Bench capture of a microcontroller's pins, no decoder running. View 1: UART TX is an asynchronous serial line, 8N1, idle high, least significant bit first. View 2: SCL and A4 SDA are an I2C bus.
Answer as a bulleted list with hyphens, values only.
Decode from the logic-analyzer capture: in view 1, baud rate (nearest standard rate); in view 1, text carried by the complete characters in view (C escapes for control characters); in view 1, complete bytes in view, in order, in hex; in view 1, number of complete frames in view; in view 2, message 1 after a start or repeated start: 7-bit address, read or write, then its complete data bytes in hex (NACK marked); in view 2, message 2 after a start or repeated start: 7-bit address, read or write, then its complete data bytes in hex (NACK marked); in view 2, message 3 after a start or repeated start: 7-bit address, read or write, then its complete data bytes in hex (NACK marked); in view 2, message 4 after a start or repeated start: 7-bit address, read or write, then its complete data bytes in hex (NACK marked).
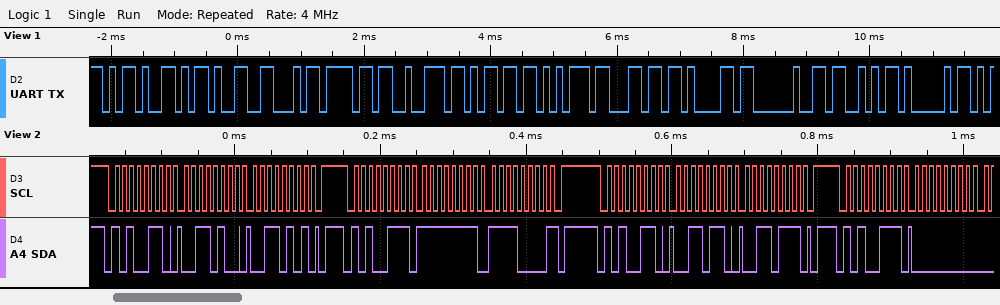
- 9600 baud
- "--Formula SA"
- 0x2D 0x2D 0x46 0x6F 0x72 0x6D 0x75 0x6C 0x61 0x20 0x53 0x41
- 12
- 0x53 write: 34 35
- 0x53 read: FF F0 NACK
- 0x53 write: 36 37
- 0x53 read: 00
